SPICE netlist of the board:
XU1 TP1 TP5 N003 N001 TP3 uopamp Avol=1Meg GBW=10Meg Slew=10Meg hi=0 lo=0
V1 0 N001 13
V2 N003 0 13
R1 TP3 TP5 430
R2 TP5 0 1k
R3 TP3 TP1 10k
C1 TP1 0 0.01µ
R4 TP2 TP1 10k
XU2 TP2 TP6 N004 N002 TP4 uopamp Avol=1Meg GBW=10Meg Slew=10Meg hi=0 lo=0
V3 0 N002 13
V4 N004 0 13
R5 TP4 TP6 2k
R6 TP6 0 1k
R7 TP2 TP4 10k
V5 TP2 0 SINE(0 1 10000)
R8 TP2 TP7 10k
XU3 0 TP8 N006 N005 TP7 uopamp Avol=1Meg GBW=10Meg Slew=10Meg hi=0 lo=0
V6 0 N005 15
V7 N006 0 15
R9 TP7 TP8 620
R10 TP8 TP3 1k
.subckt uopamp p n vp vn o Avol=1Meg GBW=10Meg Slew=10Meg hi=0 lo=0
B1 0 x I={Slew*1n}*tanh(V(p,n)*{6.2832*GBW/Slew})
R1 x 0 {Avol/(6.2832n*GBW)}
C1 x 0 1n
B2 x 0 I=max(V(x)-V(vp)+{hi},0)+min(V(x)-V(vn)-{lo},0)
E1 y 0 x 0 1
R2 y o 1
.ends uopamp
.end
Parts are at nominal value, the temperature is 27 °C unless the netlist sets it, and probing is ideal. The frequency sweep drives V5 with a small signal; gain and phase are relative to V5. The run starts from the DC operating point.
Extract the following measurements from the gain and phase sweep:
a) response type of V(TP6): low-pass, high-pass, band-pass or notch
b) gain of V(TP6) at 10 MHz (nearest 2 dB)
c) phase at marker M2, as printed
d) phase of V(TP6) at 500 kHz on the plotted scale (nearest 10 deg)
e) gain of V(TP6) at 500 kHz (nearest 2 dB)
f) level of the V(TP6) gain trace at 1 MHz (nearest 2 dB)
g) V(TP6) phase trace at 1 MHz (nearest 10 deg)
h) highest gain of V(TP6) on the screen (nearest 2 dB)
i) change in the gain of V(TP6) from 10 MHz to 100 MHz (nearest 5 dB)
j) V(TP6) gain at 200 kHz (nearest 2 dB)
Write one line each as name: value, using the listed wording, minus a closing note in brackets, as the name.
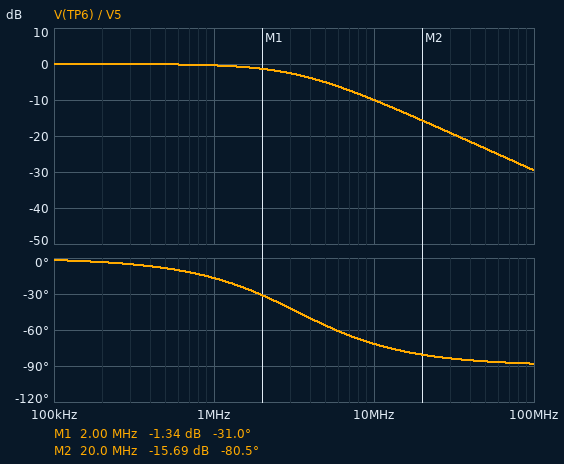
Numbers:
response type of V(TP6): low-pass, high-pass, band-pass or notch: low-pass
gain of V(TP6) at 10 MHz: -10 dB
phase at marker M2, as printed: -80.5 deg
phase of V(TP6) at 500 kHz on the plotted scale: -10 deg
gain of V(TP6) at 500 kHz: 0 dB
level of the V(TP6) gain trace at 1 MHz: 0 dB
V(TP6) phase trace at 1 MHz: -20 deg
highest gain of V(TP6) on the screen: 0 dB
change in the gain of V(TP6) from 10 MHz to 100 MHz: -20 dB
V(TP6) gain at 200 kHz: 0 dB
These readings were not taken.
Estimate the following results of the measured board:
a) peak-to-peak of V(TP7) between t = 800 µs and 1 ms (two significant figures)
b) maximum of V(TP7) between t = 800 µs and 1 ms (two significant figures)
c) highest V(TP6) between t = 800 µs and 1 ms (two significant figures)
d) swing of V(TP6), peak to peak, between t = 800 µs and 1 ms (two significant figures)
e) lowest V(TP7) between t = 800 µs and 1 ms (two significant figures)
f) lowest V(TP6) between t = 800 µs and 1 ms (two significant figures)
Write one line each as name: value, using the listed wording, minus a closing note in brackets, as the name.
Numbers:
peak-to-peak of V(TP7) between t = 800 µs and 1 ms: 280 mV
maximum of V(TP7) between t = 800 µs and 1 ms: 140 mV
highest V(TP6) between t = 800 µs and 1 ms: 1.0 V
swing of V(TP6), peak to peak, between t = 800 µs and 1 ms: 2.0 V
lowest V(TP7) between t = 800 µs and 1 ms: -140 mV
lowest V(TP6) between t = 800 µs and 1 ms: -1.0 V
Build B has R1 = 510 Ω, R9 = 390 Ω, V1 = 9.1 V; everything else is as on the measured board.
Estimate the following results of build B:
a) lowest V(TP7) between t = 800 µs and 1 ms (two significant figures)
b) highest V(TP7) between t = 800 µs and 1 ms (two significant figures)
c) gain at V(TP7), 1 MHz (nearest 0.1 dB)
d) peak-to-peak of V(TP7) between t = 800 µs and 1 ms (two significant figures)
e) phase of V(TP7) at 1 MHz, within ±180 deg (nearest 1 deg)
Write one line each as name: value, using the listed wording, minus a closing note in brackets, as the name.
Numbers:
lowest V(TP7) between t = 800 µs and 1 ms: -95 mV
highest V(TP7) between t = 800 µs and 1 ms: 93 mV
gain at V(TP7), 1 MHz: -60.6 dB
peak-to-peak of V(TP7) between t = 800 µs and 1 ms: 190 mV
phase of V(TP7) at 1 MHz, within ±180 deg: 74 deg
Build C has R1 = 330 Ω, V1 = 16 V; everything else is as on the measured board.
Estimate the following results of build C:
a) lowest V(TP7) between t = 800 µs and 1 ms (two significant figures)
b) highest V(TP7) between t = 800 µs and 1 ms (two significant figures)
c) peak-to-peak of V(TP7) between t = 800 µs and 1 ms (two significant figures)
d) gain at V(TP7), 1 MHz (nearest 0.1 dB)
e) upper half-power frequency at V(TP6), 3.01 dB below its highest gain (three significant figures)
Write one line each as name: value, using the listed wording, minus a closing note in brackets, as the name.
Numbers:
lowest V(TP7) between t = 800 µs and 1 ms: -130 mV
highest V(TP7) between t = 800 µs and 1 ms: 130 mV
peak-to-peak of V(TP7) between t = 800 µs and 1 ms: 260 mV
gain at V(TP7), 1 MHz: -57.7 dB
upper half-power frequency at V(TP6), 3.01 dB below its highest gain: 3.33 MHz
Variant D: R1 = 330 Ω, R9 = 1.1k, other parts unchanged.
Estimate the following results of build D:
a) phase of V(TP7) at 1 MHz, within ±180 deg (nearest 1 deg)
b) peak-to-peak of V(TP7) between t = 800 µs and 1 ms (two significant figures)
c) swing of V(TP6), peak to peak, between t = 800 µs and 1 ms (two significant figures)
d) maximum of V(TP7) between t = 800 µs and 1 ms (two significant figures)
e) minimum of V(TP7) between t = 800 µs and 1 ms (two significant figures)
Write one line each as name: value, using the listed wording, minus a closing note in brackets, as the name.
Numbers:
phase of V(TP7) at 1 MHz, within ±180 deg: 71 deg
peak-to-peak of V(TP7) between t = 800 µs and 1 ms: 460 mV
swing of V(TP6), peak to peak, between t = 800 µs and 1 ms: 2.0 V
maximum of V(TP7) between t = 800 µs and 1 ms: 230 mV
minimum of V(TP7) between t = 800 µs and 1 ms: -230 mV
